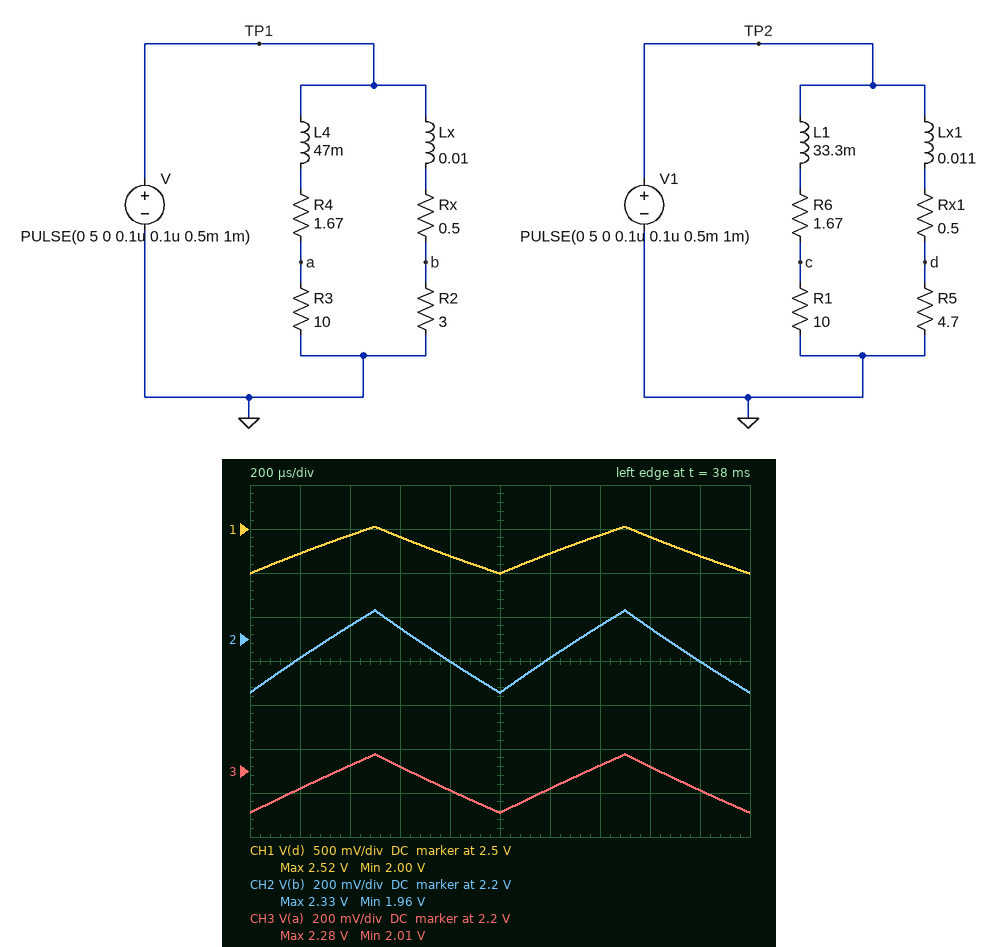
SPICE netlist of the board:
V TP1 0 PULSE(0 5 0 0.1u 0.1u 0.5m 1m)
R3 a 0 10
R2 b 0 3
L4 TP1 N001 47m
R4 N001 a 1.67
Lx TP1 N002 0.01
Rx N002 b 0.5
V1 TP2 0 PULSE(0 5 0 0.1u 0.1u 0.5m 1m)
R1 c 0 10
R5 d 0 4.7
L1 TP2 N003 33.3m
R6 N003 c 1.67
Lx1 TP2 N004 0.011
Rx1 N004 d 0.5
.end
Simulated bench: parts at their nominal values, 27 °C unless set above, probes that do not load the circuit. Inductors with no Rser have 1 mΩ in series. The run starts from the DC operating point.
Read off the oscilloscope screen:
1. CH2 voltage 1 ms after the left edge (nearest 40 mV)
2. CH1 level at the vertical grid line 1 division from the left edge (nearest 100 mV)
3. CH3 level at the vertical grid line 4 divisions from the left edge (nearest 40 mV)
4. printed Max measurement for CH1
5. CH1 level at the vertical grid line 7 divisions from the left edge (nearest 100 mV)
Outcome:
1.96 V
2.2 V
2.12 V
2.52 V
2.4 V
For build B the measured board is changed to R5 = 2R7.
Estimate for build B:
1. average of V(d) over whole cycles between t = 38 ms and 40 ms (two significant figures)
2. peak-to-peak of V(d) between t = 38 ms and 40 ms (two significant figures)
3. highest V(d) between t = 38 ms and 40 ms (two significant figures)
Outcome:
2.1 V
310 mV
2.3 V
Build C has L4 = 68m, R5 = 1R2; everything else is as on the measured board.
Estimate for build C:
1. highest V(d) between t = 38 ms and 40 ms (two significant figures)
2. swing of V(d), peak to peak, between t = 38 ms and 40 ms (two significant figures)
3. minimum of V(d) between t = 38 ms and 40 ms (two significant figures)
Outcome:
1.8 V
140 mV
1.7 V
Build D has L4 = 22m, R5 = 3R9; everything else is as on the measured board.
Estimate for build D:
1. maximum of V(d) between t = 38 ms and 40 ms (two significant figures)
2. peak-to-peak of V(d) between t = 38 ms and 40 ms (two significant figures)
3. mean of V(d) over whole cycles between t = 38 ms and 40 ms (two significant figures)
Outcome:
2.4 V
440 mV
2.2 V
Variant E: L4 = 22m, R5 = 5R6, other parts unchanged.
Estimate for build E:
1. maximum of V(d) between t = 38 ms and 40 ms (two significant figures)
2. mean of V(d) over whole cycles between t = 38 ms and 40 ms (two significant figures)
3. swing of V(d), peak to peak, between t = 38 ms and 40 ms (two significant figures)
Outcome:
2.6 V
2.3 V
630 mV
